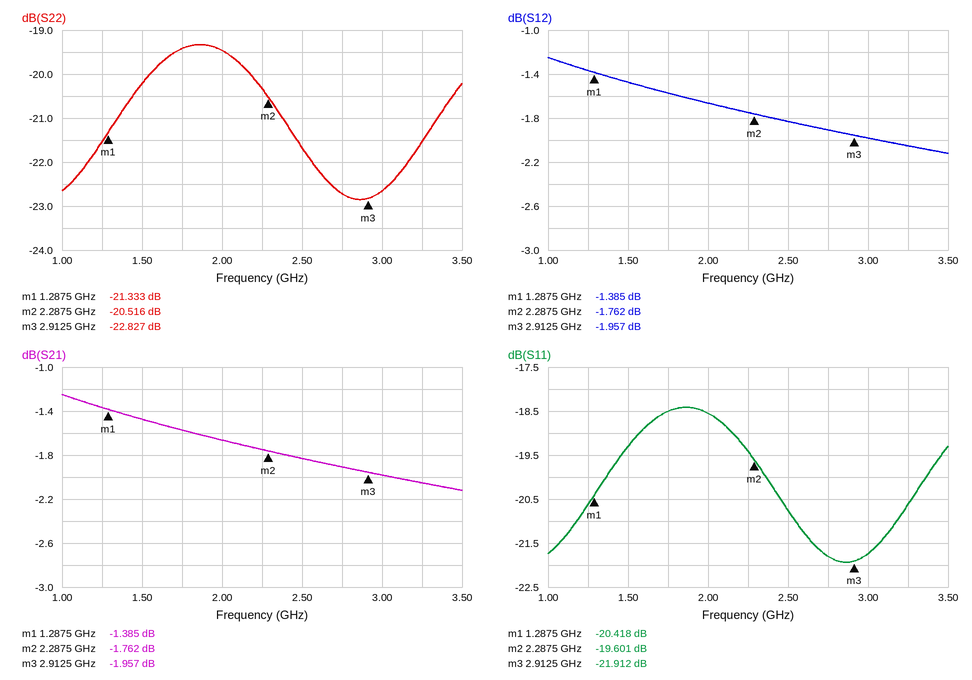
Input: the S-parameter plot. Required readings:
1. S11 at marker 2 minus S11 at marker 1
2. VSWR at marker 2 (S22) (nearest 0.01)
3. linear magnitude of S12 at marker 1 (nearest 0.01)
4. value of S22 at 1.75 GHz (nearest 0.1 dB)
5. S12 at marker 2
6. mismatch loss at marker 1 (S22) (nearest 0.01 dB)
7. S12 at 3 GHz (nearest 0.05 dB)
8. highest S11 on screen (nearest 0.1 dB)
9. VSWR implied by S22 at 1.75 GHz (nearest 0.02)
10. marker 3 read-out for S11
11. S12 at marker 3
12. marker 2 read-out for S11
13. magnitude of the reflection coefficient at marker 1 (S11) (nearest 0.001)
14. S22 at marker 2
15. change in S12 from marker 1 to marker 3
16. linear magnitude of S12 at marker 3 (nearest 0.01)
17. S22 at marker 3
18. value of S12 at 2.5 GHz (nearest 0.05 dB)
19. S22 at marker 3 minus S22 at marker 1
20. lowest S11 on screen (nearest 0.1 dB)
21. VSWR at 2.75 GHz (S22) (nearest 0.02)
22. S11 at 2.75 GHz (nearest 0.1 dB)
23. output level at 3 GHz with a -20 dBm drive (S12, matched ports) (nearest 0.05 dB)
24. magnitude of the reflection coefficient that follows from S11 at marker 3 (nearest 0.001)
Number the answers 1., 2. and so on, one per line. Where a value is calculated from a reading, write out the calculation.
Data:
1. -19.601 − (-20.418) = 0.817 dB
2. (1 + 0.0942)/(1 − 0.0942) ≈ 1.21
3. 10^(-1.385/20) ≈ 0.85
4. -19.4 dB
5. -1.762 dB
6. −10 log10(1 − 10^(-21.333/10)) ≈ 0.03 dB
7. -2.00 dB
8. -18.4 dB
9. |Γ| = 10^(-19.4/20) = 0.1072; VSWR = (1 + 0.1072)/(1 − 0.1072) ≈ 1.24
10. -21.912 dB
11. -1.957 dB
12. -19.601 dB
13. 10^(-20.418/20) ≈ 0.095
14. -20.516 dB
15. -1.957 − (-1.385) = -0.572 dB
16. 10^(-1.957/20) ≈ 0.80
17. -22.827 dB
18. -1.85 dB
19. -22.827 − (-21.333) = -1.494 dB
20. -21.9 dB
21. |Γ| = 10^(-22.7/20) = 0.0733; VSWR = (1 + 0.0733)/(1 − 0.0733) ≈ 1.16
22. -21.8 dB
23. -20 dBm + (-2.00 dB) = -22.00 dBm
24. 10^(-21.912/20) ≈ 0.080
